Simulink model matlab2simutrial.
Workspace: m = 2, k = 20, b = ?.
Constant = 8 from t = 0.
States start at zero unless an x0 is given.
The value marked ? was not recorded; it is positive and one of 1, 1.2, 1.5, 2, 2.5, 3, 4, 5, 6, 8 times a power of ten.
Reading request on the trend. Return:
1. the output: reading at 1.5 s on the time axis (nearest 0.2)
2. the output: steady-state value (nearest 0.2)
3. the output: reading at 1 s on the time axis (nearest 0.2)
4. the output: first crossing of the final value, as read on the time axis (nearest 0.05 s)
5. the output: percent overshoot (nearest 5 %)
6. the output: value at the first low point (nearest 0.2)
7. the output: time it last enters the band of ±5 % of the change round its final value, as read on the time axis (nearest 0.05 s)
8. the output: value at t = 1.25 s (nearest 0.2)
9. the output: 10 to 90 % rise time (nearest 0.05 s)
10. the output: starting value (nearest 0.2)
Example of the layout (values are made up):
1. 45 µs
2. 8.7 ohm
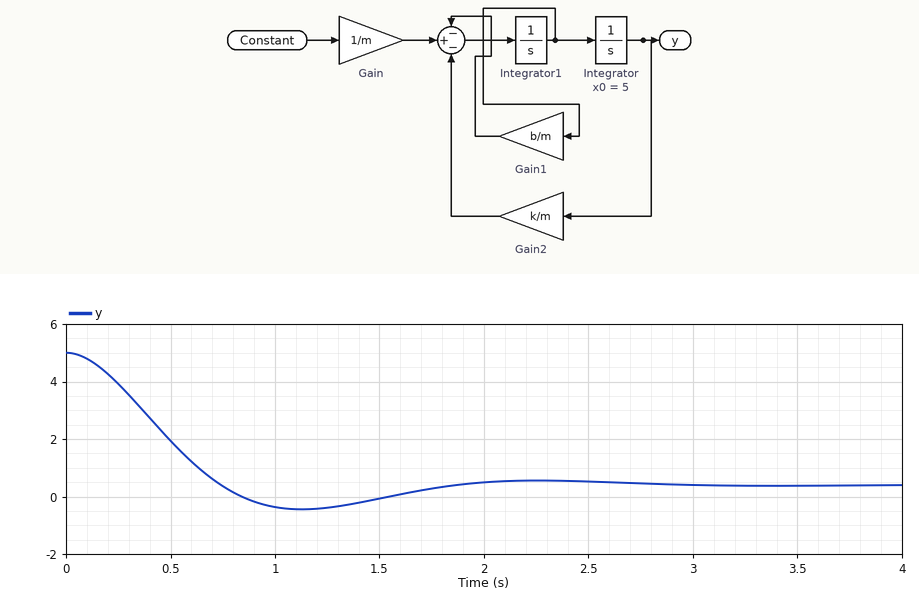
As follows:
1. 0.0
2. 0.4
3. -0.4
4. 0.75 s
5. 20 %
6. -0.4
7. 1.65 s
8. -0.4
9. 0.50 s
10. 5.0
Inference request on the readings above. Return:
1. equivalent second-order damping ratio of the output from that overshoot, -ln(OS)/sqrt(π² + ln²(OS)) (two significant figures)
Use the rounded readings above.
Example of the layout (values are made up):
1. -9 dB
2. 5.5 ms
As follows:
1. 0.46
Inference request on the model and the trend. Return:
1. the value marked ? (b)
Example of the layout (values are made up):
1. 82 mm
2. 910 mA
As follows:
1. 6
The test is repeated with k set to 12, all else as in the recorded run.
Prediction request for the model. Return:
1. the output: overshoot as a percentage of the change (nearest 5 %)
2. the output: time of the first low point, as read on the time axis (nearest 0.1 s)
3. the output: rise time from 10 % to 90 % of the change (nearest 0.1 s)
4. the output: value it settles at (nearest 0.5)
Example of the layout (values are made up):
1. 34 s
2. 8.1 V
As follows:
1. 10 %
2. 1.6 s
3. 0.8 s
4. 0.5
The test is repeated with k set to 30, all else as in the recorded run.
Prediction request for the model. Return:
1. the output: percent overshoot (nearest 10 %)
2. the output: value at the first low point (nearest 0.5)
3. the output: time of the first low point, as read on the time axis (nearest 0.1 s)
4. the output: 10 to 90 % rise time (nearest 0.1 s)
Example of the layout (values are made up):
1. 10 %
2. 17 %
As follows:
1. 30 %
2. -1.0
3. 0.9 s
4. 0.4 s
